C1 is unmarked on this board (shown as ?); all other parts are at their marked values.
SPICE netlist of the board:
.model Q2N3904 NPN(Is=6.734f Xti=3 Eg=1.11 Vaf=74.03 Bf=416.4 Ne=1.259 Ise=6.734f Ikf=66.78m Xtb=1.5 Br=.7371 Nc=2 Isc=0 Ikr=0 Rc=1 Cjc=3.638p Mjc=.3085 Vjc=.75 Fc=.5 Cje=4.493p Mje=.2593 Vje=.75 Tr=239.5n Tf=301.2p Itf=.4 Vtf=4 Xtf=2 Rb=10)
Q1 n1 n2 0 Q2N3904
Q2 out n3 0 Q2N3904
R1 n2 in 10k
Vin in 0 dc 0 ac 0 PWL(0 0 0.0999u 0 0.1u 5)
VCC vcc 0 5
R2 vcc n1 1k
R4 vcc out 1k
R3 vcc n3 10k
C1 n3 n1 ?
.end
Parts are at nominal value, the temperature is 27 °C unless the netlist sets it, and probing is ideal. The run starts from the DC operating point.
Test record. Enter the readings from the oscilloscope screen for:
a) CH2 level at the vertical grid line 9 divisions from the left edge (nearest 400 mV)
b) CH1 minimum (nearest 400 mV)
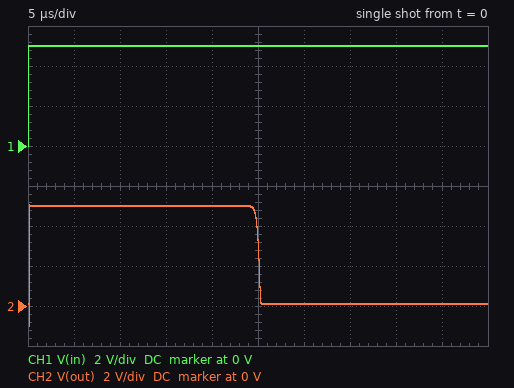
0 V
0 V
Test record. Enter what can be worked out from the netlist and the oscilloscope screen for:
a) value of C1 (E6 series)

3.3 nF
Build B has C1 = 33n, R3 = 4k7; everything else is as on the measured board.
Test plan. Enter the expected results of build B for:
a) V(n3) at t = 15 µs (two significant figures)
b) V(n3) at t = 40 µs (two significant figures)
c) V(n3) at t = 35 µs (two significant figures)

-3.3 V
-2.1 V
-2.3 V
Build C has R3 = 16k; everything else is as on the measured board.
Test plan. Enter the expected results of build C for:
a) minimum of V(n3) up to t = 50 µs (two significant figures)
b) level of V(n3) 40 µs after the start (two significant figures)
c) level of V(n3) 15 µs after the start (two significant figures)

-4.1 V
680 mV
-1.9 V
